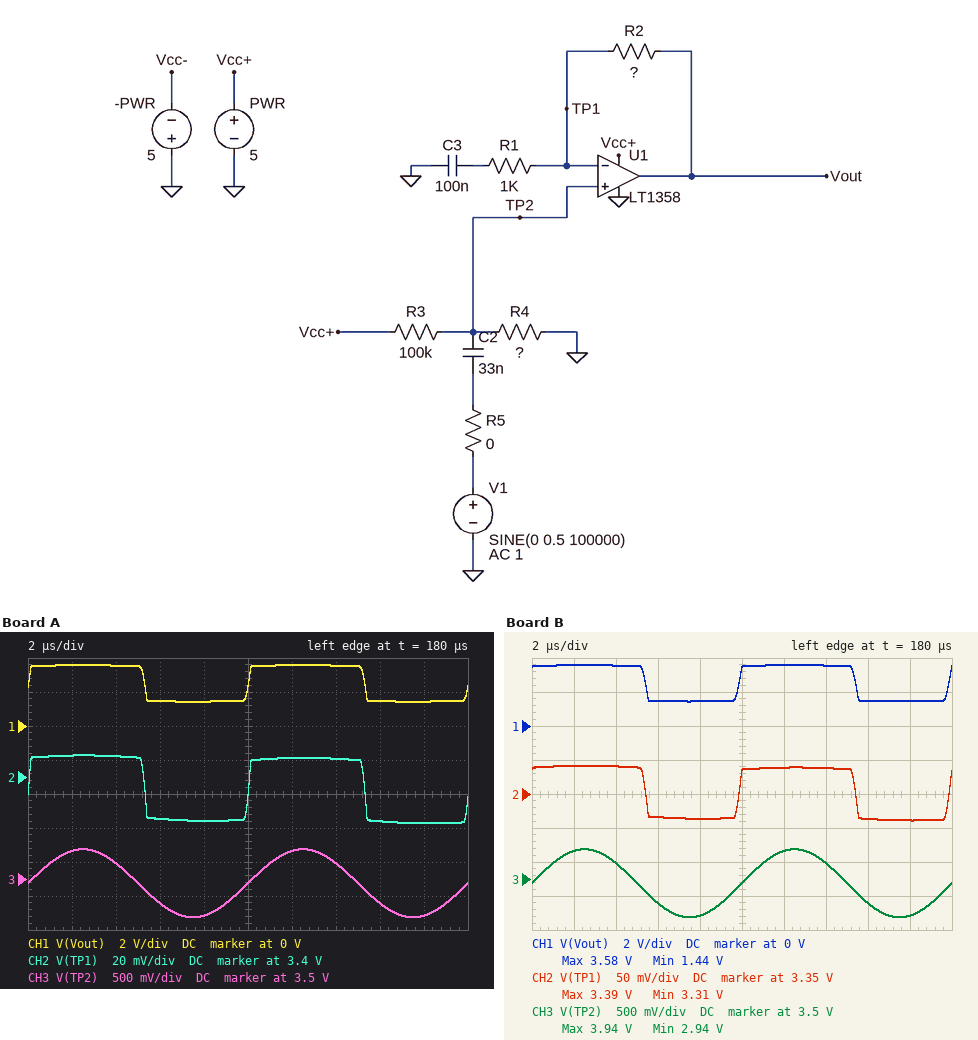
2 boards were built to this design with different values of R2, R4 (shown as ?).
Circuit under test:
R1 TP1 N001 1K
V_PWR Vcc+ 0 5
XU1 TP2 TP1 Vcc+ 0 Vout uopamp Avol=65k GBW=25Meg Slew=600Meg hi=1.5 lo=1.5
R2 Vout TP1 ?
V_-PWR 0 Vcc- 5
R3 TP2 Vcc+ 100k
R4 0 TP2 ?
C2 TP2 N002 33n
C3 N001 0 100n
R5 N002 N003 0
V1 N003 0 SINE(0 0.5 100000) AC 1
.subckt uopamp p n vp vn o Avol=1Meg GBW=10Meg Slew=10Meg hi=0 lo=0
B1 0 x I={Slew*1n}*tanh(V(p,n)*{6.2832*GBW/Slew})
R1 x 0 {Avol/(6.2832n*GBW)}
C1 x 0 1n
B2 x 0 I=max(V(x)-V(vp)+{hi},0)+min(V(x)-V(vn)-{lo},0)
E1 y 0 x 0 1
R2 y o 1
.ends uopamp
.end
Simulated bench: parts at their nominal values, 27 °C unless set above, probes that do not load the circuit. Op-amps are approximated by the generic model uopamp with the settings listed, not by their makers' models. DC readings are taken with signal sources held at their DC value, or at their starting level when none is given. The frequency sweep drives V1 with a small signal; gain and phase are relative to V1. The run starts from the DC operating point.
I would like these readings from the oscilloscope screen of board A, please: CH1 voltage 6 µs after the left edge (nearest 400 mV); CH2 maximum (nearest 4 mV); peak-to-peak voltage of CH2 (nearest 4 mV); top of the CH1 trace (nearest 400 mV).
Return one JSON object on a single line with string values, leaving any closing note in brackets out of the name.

{"CH1 voltage 6 µs after the left edge": "1.6 V", "CH2 maximum": "3.412 V", "peak-to-peak voltage of CH2": "40 mV", "top of the CH1 trace": "3.6 V"}
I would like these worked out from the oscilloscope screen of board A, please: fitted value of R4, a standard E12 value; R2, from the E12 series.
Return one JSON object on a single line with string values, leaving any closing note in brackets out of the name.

{"fitted value of R4, a standard E12 value": "220 kΩ", "R2, from the E12 series": "56 kΩ"}
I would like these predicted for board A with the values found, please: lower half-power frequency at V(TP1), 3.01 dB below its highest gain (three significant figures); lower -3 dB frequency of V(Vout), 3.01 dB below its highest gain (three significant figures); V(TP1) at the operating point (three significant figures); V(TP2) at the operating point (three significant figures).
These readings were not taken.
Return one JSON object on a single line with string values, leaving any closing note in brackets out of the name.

{"lower half-power frequency at V(TP1), 3.01 dB below its highest gain": "70.5 Hz", "lower -3 dB frequency of V(Vout), 3.01 dB below its highest gain": "1.59 kHz", "V(TP1) at the operating point": "3.44 V", "V(TP2) at the operating point": "3.44 V"}
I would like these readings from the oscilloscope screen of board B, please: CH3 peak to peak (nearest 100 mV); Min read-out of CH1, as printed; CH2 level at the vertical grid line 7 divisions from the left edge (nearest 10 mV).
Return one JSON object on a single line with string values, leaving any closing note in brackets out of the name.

{"CH3 peak to peak": "1.0 V", "Min read-out of CH1, as printed": "1.44 V", "CH2 level at the vertical grid line 7 divisions from the left edge": "3.39 V"}
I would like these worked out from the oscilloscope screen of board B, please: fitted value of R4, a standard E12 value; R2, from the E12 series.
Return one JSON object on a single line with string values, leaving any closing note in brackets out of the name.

{"fitted value of R4, a standard E12 value": "220 kΩ", "R2, from the E12 series": "27 kΩ"}
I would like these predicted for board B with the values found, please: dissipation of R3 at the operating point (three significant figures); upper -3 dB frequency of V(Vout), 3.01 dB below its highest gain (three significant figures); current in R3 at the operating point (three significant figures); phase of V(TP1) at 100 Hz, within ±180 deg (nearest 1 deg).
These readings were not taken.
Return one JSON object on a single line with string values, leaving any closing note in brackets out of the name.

{"dissipation of R3 at the operating point": "24.4 µW", "upper -3 dB frequency of V(Vout), 3.01 dB below its highest gain": "895 kHz", "current in R3 at the operating point": "15.6 µA", "phase of V(TP1) at 100 Hz, within ±180 deg": "35 deg"}
